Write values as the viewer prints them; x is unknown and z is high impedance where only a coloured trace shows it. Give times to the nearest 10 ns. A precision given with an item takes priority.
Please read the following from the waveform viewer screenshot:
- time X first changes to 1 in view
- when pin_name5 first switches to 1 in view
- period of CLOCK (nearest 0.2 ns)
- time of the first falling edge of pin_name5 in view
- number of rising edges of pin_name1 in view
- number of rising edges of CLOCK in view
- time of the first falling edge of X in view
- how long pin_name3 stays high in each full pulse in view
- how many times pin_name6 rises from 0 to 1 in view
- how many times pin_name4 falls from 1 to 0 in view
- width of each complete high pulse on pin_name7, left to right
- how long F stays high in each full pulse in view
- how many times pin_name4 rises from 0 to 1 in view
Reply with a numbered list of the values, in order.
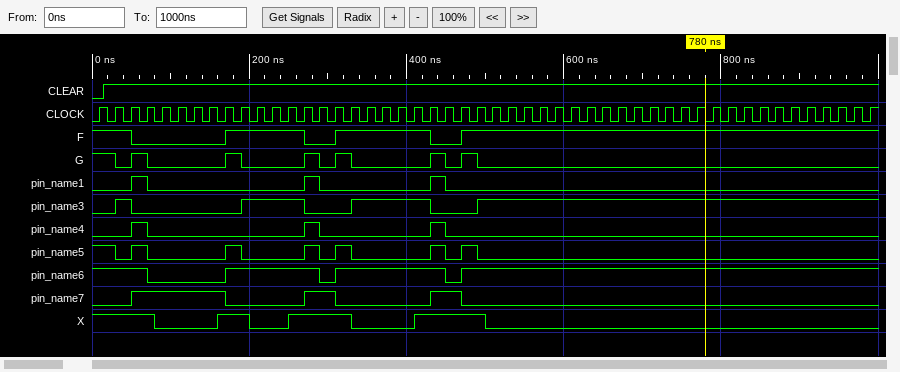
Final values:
1. 160 ns
2. 50 ns
3. 20 ns
4. 30 ns
5. 3
6. 50
7. 80 ns
8. 20 ns, 80 ns, 100 ns
9. 3
10. 3
11. 120 ns, 40 ns, 40 ns
12. 100 ns, 120 ns
13. 3
